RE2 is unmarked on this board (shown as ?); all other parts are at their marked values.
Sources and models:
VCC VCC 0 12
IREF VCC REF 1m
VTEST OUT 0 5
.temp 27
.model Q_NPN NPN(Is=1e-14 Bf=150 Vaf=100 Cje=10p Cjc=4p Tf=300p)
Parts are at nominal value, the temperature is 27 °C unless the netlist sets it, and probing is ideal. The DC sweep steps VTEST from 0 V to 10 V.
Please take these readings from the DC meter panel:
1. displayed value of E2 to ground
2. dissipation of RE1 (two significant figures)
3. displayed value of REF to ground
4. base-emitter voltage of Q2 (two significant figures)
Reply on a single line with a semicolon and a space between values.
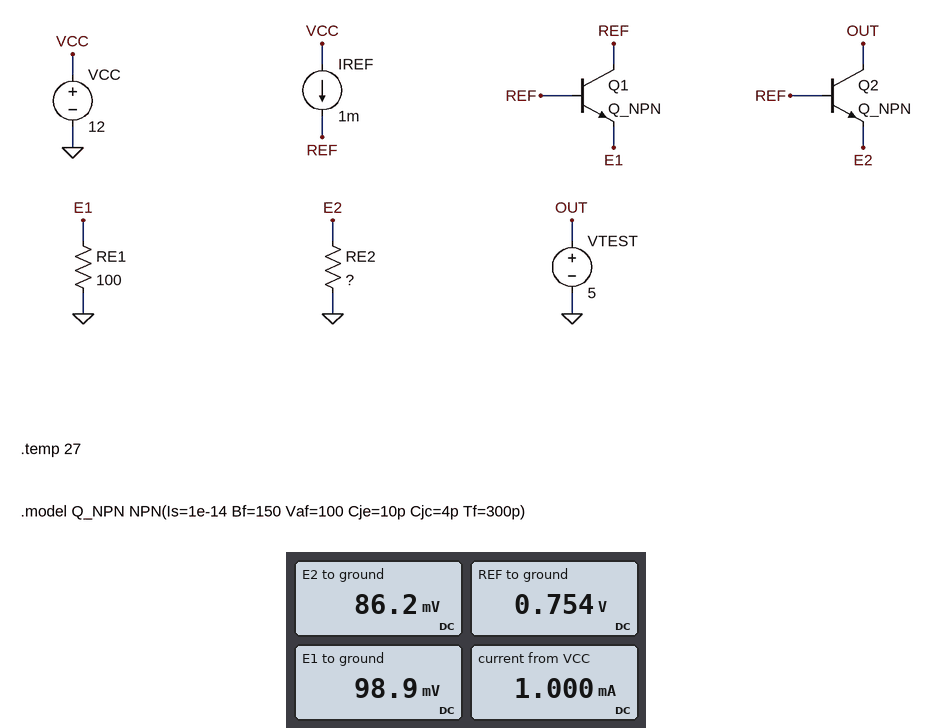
86.2 mV; 98 µW; 0.754 V; 670 mV
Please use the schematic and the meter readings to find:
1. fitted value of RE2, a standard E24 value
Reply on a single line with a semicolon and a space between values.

51 Ω
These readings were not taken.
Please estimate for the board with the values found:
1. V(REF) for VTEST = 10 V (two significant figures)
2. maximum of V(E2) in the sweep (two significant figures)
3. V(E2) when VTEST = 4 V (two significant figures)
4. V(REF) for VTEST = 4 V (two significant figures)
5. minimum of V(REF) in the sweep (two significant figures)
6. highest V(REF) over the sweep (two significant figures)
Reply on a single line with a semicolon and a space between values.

750 mV; 87 mV; 86 mV; 750 mV; 650 mV; 750 mV
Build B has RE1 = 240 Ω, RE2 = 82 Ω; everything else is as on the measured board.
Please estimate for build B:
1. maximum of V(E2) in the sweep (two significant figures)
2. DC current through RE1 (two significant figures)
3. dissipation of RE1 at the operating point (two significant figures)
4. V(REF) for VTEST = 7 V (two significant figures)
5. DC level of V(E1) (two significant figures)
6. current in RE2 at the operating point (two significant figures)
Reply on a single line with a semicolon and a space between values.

210 mV; 980 µA; 230 µW; 890 mV; 240 mV; 2.6 mA
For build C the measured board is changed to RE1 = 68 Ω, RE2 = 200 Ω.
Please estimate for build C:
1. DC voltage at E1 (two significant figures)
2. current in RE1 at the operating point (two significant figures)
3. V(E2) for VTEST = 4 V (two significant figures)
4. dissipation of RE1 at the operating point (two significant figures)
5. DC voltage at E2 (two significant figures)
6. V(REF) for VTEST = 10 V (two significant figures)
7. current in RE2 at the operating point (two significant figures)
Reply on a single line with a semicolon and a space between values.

68 mV; 1.0 mA; 89 mV; 68 µW; 90 mV; 720 mV; 450 µA
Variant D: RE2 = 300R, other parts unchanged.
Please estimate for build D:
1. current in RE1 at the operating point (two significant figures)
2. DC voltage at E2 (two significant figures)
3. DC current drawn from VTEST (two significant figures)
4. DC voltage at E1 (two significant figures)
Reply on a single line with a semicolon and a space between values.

1.0 mA; 120 mV; 410 µA; 100 mV
